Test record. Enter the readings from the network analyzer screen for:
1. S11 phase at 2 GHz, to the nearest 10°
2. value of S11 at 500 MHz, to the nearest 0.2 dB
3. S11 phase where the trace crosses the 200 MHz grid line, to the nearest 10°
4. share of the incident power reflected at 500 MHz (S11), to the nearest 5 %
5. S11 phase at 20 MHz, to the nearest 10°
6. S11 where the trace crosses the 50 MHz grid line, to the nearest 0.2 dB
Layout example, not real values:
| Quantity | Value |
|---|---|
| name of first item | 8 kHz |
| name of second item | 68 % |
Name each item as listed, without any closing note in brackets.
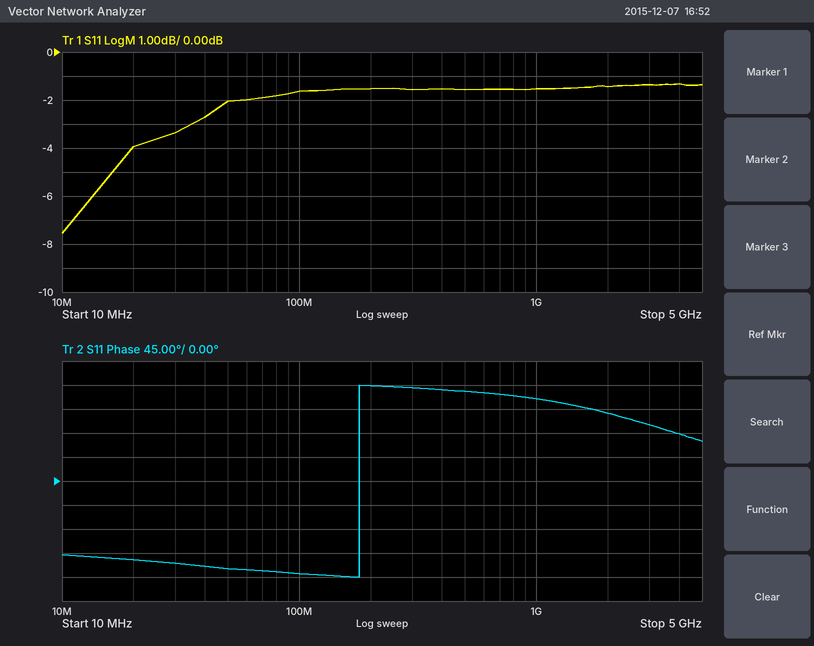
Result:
| Quantity | Value |
|---|---|
| S11 phase at 2 GHz, to the nearest 10° | 130° |
| value of S11 at 500 MHz, to the nearest 0.2 dB | -1.6 dB |
| S11 phase where the trace crosses the 200 MHz grid line, to the nearest 10° | 180° |
| share of the incident power reflected at 500 MHz (S11), to the nearest 5 % | 70 % |
| S11 phase at 20 MHz, to the nearest 10° | -150° |
| S11 where the trace crosses the 50 MHz grid line, to the nearest 0.2 dB | -2.0 dB |
